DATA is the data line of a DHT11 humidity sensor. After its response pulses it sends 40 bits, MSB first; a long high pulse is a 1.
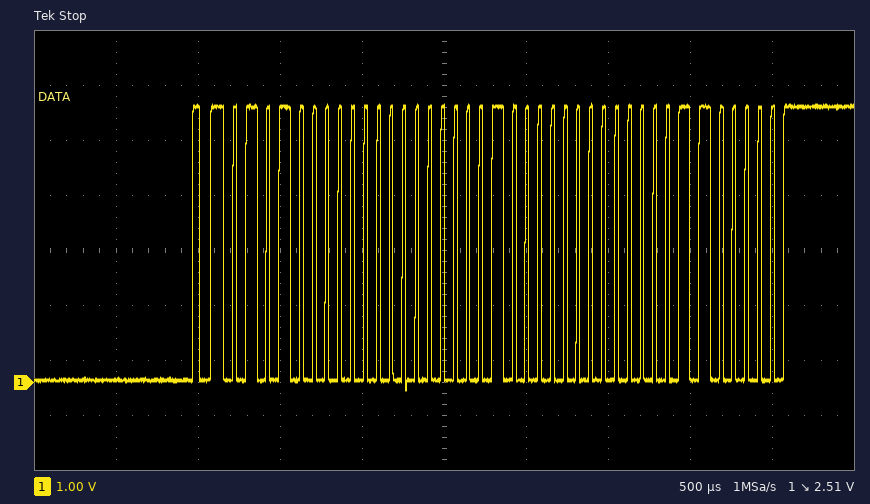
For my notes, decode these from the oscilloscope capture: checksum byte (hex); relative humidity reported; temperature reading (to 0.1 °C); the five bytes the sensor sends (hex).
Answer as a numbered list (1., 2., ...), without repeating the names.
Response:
1. 0x60
2. 80 %
3. 16.0 °C
4. 50 00 10 00 60
